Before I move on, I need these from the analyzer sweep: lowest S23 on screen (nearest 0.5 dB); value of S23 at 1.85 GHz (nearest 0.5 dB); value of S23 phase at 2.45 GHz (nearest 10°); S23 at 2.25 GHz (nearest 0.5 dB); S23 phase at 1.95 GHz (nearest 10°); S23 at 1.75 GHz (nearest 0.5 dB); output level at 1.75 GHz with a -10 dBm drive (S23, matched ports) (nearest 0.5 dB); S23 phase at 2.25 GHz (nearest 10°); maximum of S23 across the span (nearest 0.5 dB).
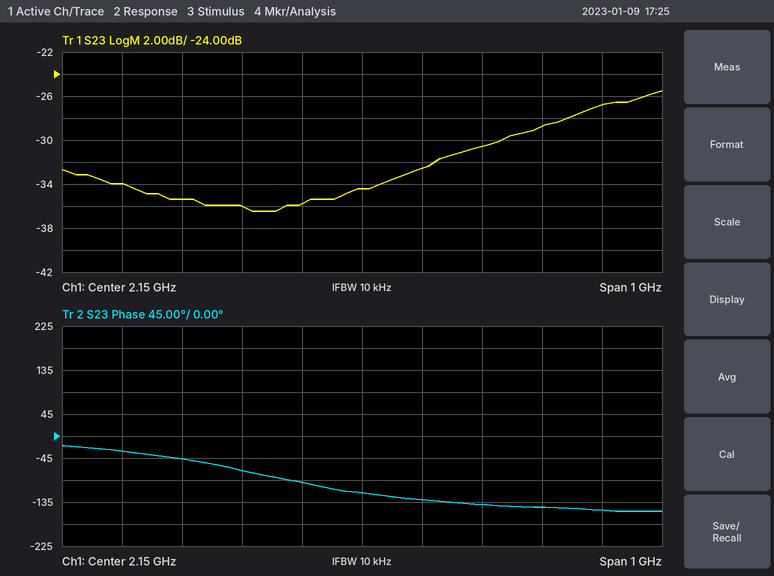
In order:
-36.5 dB
-35.5 dB
-150°
-32.5 dB
-70°
-34.0 dB
-44.0 dBm
-130°
-25.5 dB
